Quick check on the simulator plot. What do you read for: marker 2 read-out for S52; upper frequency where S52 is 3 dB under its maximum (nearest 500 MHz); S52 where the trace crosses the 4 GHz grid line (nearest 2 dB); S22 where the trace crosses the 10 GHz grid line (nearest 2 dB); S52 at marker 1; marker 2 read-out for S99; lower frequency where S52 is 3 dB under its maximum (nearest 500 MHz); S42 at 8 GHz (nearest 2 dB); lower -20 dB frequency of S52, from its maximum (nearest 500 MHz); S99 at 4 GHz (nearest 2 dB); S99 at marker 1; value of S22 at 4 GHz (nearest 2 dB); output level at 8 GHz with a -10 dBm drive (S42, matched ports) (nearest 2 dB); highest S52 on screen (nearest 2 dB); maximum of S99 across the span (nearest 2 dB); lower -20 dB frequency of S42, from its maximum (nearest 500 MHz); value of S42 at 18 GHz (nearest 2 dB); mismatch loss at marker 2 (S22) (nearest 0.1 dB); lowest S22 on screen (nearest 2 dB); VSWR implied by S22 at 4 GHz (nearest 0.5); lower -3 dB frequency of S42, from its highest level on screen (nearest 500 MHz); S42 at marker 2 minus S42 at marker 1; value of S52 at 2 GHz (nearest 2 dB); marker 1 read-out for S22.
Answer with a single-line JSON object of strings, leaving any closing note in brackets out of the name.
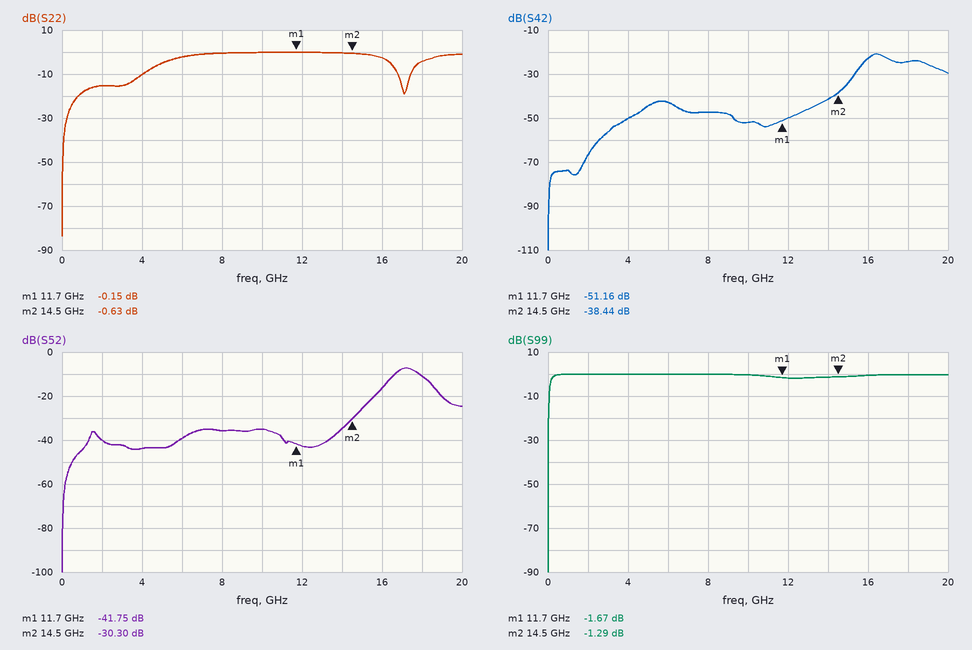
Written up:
{"marker 2 read-out for S52": "-30.30 dB", "upper frequency where S52 is 3 dB under its maximum": "18.0 GHz", "S52 where the trace crosses the 4 GHz grid line": "-44 dB", "S22 where the trace crosses the 10 GHz grid line": "0 dB", "S52 at marker 1": "-41.75 dB", "marker 2 read-out for S99": "-1.29 dB", "lower frequency where S52 is 3 dB under its maximum": "16.5 GHz", "S42 at 8 GHz": "-48 dB", "lower -20 dB frequency of S52, from its maximum": "15.0 GHz", "S99 at 4 GHz": "0 dB", "S99 at marker 1": "-1.67 dB", "value of S22 at 4 GHz": "-10 dB", "output level at 8 GHz with a -10 dBm drive (S42, matched ports)": "-58 dBm", "highest S52 on screen": "-8 dB", "maximum of S99 across the span": "0 dB", "lower -20 dB frequency of S42, from its maximum": "14.0 GHz", "value of S42 at 18 GHz": "-24 dB", "mismatch loss at marker 2 (S22)": "8.7 dB", "lowest S22 on screen": "-84 dB", "VSWR implied by S22 at 4 GHz": "2.0", "lower -3 dB frequency of S42, from its highest level on screen": "16.0 GHz", "S42 at marker 2 minus S42 at marker 1": "12.72 dB", "value of S52 at 2 GHz": "-40 dB", "marker 1 read-out for S22": "-0.15 dB"}
